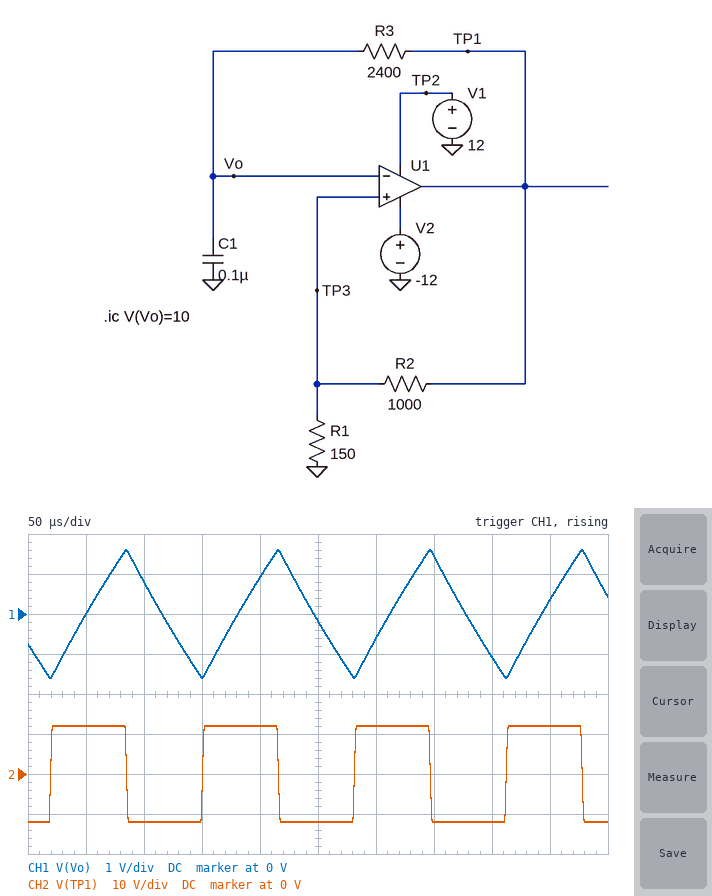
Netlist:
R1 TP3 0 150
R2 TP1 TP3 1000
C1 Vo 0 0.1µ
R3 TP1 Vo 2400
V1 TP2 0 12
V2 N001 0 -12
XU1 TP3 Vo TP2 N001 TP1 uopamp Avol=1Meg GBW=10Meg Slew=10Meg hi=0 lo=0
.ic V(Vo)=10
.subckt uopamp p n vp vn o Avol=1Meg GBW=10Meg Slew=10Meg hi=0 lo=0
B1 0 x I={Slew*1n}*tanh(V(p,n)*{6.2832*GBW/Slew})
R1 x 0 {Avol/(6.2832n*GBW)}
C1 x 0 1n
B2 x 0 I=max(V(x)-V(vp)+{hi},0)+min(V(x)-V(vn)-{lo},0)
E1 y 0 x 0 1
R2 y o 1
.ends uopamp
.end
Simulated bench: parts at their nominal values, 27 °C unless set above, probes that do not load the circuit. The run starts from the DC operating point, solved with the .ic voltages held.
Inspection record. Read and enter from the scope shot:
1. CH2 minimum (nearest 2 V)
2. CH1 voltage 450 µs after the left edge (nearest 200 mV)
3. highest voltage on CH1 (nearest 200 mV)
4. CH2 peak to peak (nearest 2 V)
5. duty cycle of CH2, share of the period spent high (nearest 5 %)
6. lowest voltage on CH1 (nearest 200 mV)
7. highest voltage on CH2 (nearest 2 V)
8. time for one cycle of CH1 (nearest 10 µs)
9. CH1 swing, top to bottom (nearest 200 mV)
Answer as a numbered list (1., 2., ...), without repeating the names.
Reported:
1. -12 V
2. 400 mV
3. 1.6 V
4. 24 V
5. 50 %
6. -1.6 V
7. 12 V
8. 130 µs
9. 3.2 V
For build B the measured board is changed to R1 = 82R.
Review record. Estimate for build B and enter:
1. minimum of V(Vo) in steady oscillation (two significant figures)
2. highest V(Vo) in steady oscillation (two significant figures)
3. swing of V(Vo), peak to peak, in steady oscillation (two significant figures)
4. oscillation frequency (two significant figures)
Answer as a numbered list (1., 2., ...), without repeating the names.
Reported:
1. -950 mV
2. 950 mV
3. 1.9 V
4. 13 kHz
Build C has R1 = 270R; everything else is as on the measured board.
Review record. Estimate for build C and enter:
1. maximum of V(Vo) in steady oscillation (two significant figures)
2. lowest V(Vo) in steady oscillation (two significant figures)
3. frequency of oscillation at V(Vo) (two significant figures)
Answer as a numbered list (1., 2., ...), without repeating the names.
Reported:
1. 2.6 V
2. -2.6 V
3. 4.7 kHz
